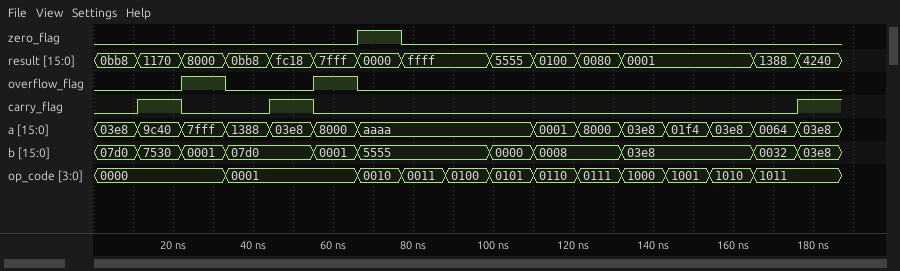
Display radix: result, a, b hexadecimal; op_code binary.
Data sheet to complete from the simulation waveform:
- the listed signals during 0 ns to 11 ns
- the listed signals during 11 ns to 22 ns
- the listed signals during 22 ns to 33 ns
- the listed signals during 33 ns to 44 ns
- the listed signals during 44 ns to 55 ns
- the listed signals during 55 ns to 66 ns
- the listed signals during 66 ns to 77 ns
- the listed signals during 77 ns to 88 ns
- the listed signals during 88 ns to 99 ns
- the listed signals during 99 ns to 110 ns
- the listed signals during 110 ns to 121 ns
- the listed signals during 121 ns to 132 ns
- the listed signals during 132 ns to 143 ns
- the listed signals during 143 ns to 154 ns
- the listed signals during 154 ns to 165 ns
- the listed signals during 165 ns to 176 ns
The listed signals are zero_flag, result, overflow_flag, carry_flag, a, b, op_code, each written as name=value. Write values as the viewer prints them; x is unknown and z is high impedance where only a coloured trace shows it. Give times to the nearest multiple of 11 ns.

zero_flag=0, result=0bb8, overflow_flag=0, carry_flag=0, a=03e8, b=07d0, op_code=0000
zero_flag=0, result=1170, overflow_flag=0, carry_flag=1, a=9c40, b=7530, op_code=0000
zero_flag=0, result=8000, overflow_flag=1, carry_flag=0, a=7fff, b=0001, op_code=0000
zero_flag=0, result=0bb8, overflow_flag=0, carry_flag=0, a=1388, b=07d0, op_code=0001
zero_flag=0, result=fc18, overflow_flag=0, carry_flag=1, a=03e8, b=07d0, op_code=0001
zero_flag=0, result=7fff, overflow_flag=1, carry_flag=0, a=8000, b=0001, op_code=0001
zero_flag=1, result=0000, overflow_flag=0, carry_flag=0, a=aaaa, b=5555, op_code=0010
zero_flag=0, result=ffff, overflow_flag=0, carry_flag=0, a=aaaa, b=5555, op_code=0011
zero_flag=0, result=ffff, overflow_flag=0, carry_flag=0, a=aaaa, b=5555, op_code=0100
zero_flag=0, result=5555, overflow_flag=0, carry_flag=0, a=aaaa, b=0000, op_code=0101
zero_flag=0, result=0100, overflow_flag=0, carry_flag=0, a=0001, b=0008, op_code=0110
zero_flag=0, result=0080, overflow_flag=0, carry_flag=0, a=8000, b=0008, op_code=0111
zero_flag=0, result=0001, overflow_flag=0, carry_flag=0, a=03e8, b=03e8, op_code=1000
zero_flag=0, result=0001, overflow_flag=0, carry_flag=0, a=01f4, b=03e8, op_code=1001
zero_flag=0, result=0001, overflow_flag=0, carry_flag=0, a=03e8, b=03e8, op_code=1010
zero_flag=0, result=1388, overflow_flag=0, carry_flag=0, a=0064, b=0032, op_code=1011
